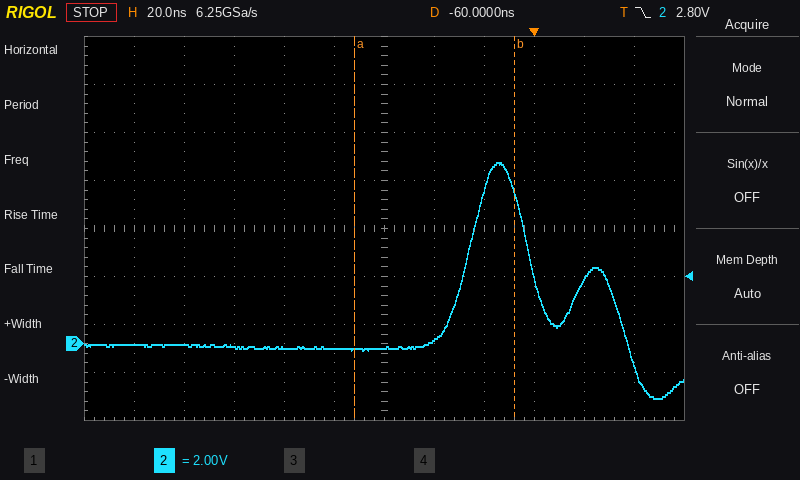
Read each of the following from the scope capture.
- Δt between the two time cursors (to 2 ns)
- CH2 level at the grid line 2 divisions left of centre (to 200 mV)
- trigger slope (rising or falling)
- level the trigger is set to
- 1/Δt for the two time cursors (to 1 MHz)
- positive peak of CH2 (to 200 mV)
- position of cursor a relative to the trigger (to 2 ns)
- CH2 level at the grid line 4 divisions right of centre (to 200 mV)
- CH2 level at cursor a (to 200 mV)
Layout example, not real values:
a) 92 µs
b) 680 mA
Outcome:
a) 64 ns
b) -200 mV
c) falling
d) 2.80 V
e) 16 MHz
f) 7.6 V
g) -72 ns
h) 2.6 V
i) -200 mV
